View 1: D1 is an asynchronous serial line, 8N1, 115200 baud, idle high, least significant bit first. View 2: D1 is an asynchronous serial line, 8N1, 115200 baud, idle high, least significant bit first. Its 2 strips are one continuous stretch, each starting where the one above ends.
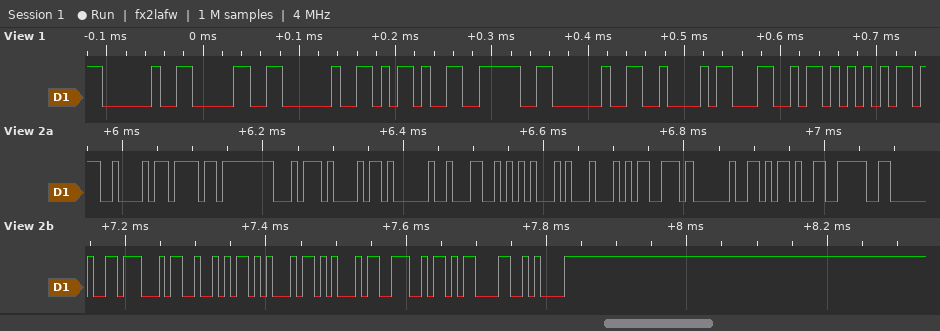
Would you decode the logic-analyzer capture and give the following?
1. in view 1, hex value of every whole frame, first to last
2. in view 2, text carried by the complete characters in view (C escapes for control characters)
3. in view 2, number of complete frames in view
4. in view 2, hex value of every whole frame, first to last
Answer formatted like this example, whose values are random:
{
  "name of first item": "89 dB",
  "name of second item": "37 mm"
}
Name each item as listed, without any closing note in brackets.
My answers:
{
  "in view 1, hex value of every whole frame, first to last": "20 30 20 2D 3E 20 42 4C 55",
  "in view 2, text carried by the complete characters in view": "\"Both LEDs -> GREEN\\r\\n\"",
  "in view 2, number of complete frames in view": "20",
  "in view 2, hex value of every whole frame, first to last": "42 6F 74 68 20 4C 45 44 73 20 2D 3E 20 47 52 45 45 4E 0D 0A"
}
